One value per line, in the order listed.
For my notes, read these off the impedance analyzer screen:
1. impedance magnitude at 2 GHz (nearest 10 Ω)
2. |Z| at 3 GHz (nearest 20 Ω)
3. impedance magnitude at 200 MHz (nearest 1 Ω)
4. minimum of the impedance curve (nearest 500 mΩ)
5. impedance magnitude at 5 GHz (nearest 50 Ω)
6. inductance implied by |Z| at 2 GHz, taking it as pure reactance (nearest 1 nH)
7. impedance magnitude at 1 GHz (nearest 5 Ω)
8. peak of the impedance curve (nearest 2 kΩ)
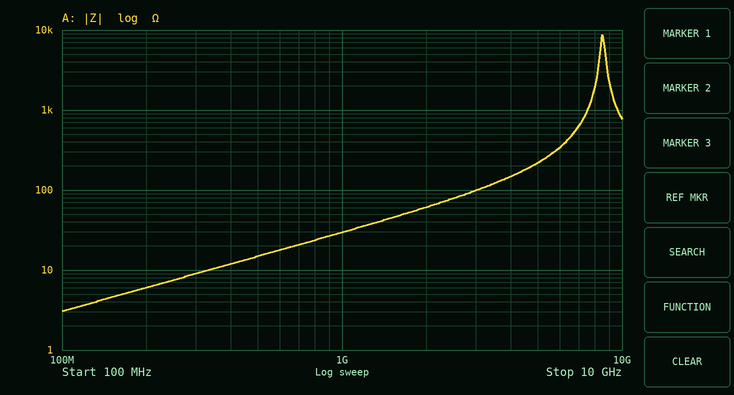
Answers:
60 Ω
100 Ω
6 Ω
3.0 Ω
200 Ω
5 nH
30 Ω
8 kΩ
